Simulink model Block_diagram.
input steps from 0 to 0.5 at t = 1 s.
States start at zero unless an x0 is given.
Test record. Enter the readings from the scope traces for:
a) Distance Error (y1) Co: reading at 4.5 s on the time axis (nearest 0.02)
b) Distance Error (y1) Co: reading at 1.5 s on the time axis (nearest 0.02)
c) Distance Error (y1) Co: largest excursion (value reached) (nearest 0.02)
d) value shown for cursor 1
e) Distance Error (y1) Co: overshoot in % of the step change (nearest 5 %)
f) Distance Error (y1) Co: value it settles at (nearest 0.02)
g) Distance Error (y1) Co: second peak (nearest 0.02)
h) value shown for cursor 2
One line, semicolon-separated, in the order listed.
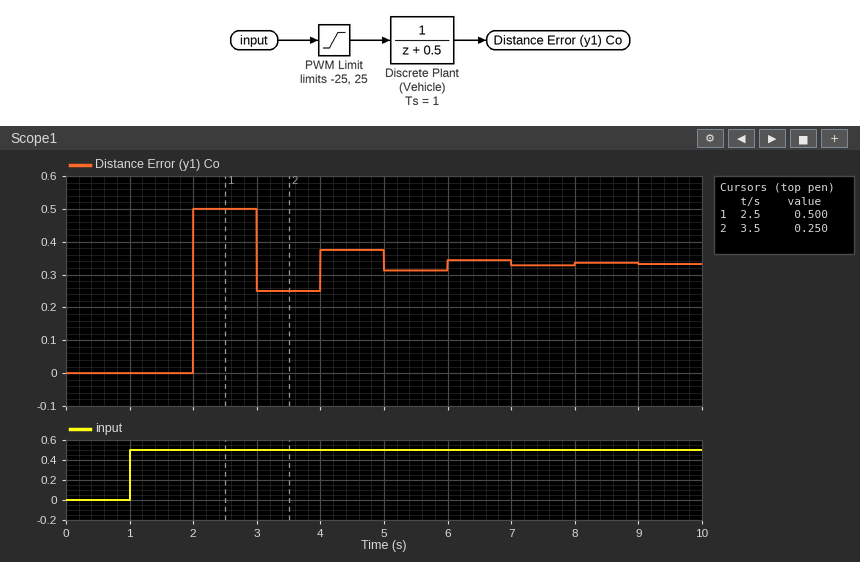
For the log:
0.38; 0.00; 0.50; 0.500; 50 %; 0.34; 0.38; 0.250
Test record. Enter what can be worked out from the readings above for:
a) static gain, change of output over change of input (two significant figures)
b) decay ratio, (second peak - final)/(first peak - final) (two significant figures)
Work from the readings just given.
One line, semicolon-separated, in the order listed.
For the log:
0.68; 0.25
